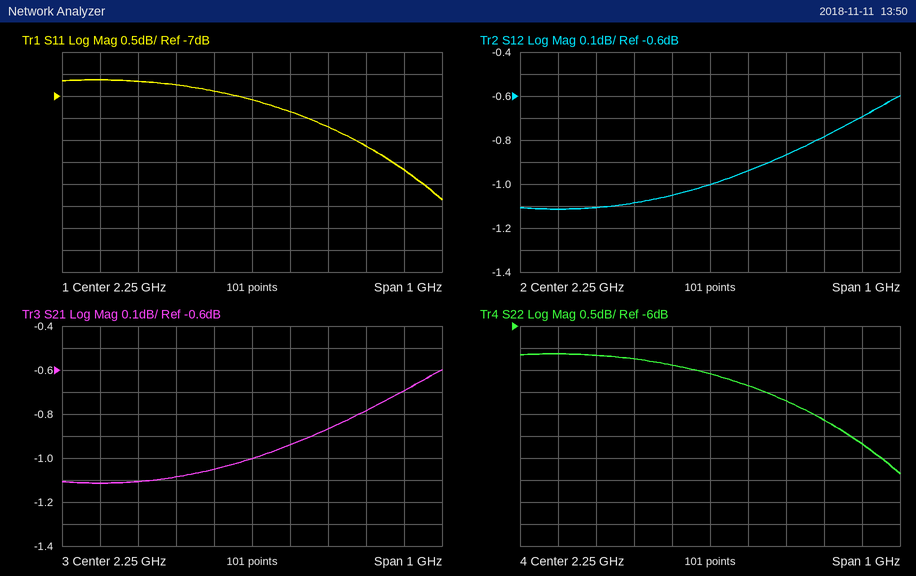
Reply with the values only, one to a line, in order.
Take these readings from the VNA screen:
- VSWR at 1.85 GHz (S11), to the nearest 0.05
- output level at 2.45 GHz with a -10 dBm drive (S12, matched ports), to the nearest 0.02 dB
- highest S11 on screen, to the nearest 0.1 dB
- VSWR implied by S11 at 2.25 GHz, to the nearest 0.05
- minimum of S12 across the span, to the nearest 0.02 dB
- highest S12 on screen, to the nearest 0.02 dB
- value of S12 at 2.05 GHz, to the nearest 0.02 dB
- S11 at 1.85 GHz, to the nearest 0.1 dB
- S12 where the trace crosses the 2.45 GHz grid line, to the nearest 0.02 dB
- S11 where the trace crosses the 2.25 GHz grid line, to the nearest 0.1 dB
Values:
2.75
-10.86 dBm
-6.6 dB
2.60
-1.12 dB
-0.60 dB
-1.08 dB
-6.6 dB
-0.86 dB
-7.1 dB
